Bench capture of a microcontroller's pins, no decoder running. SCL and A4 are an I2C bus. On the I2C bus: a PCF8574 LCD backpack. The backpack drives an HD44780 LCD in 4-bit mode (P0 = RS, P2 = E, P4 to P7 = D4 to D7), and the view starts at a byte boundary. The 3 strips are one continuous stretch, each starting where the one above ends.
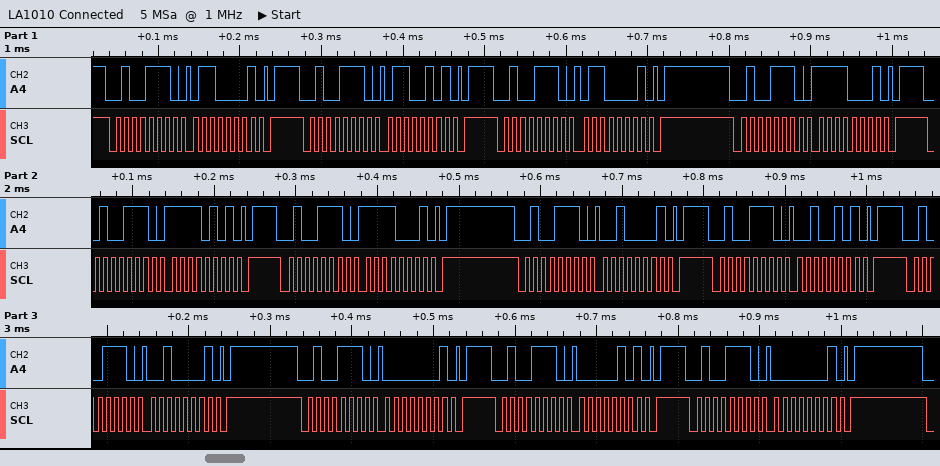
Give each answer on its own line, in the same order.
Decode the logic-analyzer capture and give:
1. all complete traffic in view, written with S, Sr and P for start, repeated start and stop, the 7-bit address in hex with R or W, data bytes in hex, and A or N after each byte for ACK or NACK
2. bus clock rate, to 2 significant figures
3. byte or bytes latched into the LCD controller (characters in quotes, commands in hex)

S 27W A 61 A P S 27W A 65 A P S 27W A 61 A P S 27W A F1 A P S 27W A F5 A P S 27W A F1 A P S 27W A 21 A P S 27W A 25 A P S 27W A 21 A P S 27W A 01 A P S 27W A 05 A P S 27W A 01 A P
100 kHz
'o' ' '
